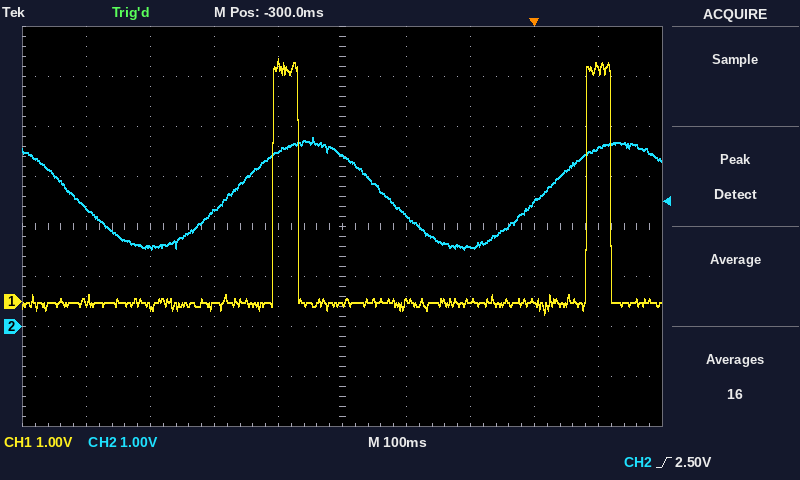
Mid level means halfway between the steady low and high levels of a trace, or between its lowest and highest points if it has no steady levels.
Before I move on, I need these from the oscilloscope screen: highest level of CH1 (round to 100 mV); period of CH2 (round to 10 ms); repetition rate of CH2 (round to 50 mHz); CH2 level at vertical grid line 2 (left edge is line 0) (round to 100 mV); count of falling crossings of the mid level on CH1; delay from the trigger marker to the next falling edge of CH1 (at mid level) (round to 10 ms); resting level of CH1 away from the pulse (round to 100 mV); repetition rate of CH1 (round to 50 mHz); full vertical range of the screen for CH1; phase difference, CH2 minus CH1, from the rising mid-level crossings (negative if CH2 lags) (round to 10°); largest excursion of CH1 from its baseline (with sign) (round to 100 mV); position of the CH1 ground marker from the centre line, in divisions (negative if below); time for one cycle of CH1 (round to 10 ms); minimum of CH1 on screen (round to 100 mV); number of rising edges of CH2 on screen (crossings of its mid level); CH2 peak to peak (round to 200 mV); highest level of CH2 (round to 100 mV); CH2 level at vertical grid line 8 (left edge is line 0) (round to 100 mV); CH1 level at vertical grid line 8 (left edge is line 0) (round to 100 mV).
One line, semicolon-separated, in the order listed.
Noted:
4.9 V; 490 ms; 2.05 Hz; 1.6 V; 2; 120 ms; 0.0 V; 2.05 Hz; 8 V; +50°; +4.9 V; -1.5 div; 490 ms; -300 mV; 2; 2.2 V; 3.8 V; 2.5 V; 0.0 V
